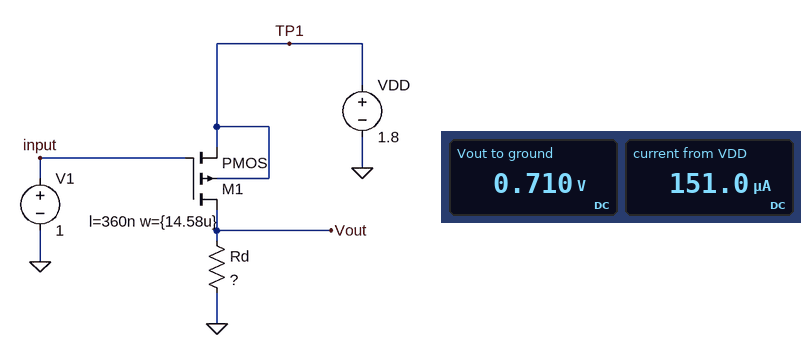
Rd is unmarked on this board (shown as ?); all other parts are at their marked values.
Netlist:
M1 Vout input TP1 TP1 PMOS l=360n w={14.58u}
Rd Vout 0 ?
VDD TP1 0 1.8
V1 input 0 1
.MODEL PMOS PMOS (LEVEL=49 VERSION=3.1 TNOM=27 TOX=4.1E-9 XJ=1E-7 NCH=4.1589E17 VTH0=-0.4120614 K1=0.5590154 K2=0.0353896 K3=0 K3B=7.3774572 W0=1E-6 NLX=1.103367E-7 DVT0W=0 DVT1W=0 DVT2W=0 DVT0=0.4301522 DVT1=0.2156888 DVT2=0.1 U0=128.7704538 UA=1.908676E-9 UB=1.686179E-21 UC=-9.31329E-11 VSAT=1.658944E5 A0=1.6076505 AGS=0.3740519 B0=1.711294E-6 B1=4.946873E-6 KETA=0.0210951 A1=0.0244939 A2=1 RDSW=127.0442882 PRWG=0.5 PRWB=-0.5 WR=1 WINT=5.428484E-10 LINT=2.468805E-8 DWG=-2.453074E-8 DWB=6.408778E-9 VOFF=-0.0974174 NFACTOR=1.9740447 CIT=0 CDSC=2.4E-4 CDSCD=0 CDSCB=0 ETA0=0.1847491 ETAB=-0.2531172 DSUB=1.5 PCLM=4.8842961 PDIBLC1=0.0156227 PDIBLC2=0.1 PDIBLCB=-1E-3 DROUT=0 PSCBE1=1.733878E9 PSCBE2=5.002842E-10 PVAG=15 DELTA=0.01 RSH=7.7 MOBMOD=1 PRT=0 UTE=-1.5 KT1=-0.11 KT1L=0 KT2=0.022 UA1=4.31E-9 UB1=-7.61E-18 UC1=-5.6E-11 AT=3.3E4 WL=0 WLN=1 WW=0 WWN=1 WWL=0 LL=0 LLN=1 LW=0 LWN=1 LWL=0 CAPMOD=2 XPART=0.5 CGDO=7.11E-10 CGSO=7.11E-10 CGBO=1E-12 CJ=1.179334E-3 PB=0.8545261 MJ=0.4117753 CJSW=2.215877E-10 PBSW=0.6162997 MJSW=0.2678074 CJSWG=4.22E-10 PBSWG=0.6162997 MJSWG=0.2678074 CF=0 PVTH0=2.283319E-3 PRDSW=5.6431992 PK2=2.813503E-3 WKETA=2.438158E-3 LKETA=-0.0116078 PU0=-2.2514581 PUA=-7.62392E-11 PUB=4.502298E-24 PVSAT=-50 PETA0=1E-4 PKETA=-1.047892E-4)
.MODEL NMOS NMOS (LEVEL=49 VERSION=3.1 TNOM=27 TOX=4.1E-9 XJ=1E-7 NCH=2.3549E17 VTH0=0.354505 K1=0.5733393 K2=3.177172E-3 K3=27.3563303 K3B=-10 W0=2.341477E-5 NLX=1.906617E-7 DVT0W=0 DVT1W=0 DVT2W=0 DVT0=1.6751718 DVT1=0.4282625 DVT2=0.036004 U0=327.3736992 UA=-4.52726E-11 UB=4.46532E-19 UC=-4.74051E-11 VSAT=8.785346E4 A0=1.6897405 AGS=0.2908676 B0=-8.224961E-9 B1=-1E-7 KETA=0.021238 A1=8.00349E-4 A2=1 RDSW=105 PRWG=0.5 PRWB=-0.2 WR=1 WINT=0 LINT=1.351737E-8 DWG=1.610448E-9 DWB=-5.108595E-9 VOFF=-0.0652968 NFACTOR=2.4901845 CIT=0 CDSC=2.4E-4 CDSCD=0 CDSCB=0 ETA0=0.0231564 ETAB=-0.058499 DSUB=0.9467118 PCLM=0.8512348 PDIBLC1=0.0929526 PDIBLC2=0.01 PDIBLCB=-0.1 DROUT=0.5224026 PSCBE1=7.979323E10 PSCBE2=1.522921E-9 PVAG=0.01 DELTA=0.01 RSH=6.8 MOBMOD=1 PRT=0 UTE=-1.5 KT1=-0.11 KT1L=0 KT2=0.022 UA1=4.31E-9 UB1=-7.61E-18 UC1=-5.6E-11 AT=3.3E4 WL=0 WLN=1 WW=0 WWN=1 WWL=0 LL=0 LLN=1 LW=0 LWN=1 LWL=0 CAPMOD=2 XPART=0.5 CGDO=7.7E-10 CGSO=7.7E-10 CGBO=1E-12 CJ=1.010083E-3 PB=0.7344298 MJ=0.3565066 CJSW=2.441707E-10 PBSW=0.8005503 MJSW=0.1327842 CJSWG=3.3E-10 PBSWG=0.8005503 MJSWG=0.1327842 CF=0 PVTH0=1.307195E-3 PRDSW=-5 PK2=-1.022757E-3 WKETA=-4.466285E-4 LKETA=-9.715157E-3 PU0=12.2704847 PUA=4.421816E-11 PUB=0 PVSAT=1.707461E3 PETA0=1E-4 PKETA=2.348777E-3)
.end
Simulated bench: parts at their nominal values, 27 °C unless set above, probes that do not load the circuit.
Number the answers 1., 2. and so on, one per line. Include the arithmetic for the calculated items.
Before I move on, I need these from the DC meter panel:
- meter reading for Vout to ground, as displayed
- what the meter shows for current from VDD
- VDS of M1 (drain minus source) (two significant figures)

1. 0.710 V
2. 151.0 µA
3. 710 mV - 1.8 V = -1.1 V
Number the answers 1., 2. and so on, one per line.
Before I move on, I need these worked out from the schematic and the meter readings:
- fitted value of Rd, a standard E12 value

1. 4.7 kΩ
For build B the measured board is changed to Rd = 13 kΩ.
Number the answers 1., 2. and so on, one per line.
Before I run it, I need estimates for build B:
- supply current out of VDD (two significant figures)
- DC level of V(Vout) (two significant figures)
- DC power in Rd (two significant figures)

1. 120 µA
2. 1.6 V
3. 200 µW
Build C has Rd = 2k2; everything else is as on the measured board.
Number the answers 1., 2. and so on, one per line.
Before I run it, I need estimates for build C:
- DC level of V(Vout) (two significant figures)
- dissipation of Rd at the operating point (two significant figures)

1. 340 mV
2. 53 µW
